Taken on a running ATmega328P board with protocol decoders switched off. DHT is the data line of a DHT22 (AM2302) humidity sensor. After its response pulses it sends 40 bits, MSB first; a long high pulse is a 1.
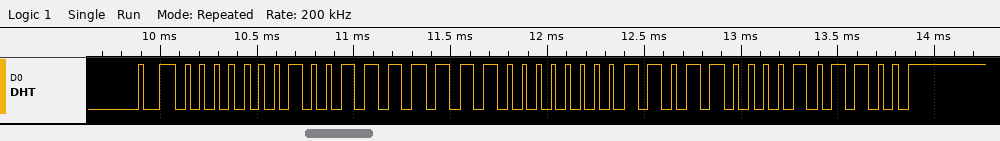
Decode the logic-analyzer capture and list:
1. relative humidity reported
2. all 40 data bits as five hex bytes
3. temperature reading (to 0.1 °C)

31.9 %
01 3F 80 6C 2C
-10.8 °C
